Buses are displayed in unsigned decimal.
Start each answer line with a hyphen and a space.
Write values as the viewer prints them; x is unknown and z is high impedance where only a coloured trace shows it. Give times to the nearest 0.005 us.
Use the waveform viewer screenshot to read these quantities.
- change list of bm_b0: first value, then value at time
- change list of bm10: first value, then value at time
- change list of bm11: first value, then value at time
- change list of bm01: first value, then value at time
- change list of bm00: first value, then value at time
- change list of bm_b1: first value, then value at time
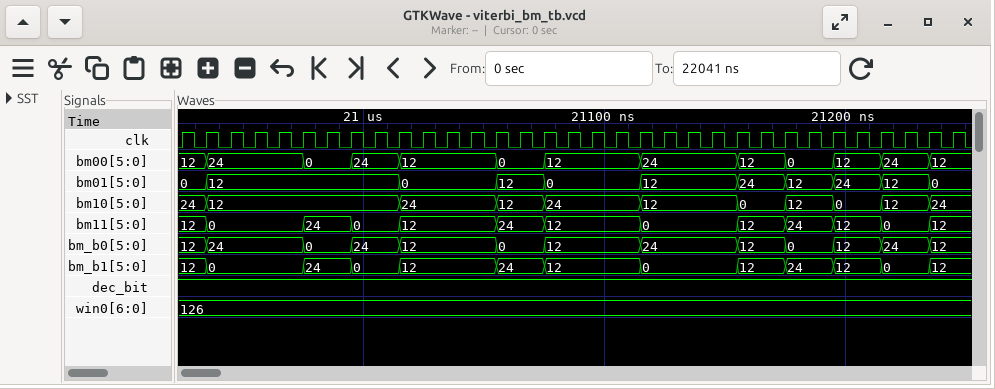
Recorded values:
- 12, 24 at 20.935 us, 0 at 20.975 us, 24 at 20.995 us, 12 at 21.015 us, 0 at 21.055 us, 12 at 21.075 us, 24 at 21.115 us, 12 at 21.155 us, 0 at 21.175 us, 12 at 21.195 us, 24 at 21.215 us, 12 at 21.235 us
- 24, 12 at 20.935 us, 24 at 21.015 us, 12 at 21.055 us, 24 at 21.075 us, 12 at 21.115 us, 0 at 21.155 us, 12 at 21.175 us, 0 at 21.195 us, 12 at 21.215 us, 24 at 21.235 us
- 12, 0 at 20.935 us, 24 at 20.975 us, 0 at 20.995 us, 12 at 21.015 us, 24 at 21.055 us, 12 at 21.075 us, 0 at 21.115 us, 12 at 21.155 us, 24 at 21.175 us, 12 at 21.195 us, 0 at 21.215 us, 12 at 21.235 us
- 0, 12 at 20.935 us, 0 at 21.015 us, 12 at 21.055 us, 0 at 21.075 us, 12 at 21.115 us, 24 at 21.155 us, 12 at 21.175 us, 24 at 21.195 us, 12 at 21.215 us, 0 at 21.235 us
- 12, 24 at 20.935 us, 0 at 20.975 us, 24 at 20.995 us, 12 at 21.015 us, 0 at 21.055 us, 12 at 21.075 us, 24 at 21.115 us, 12 at 21.155 us, 0 at 21.175 us, 12 at 21.195 us, 24 at 21.215 us, 12 at 21.235 us
- 12, 0 at 20.935 us, 24 at 20.975 us, 0 at 20.995 us, 12 at 21.015 us, 24 at 21.055 us, 12 at 21.075 us, 0 at 21.115 us, 12 at 21.155 us, 24 at 21.175 us, 12 at 21.195 us, 0 at 21.215 us, 12 at 21.235 us
